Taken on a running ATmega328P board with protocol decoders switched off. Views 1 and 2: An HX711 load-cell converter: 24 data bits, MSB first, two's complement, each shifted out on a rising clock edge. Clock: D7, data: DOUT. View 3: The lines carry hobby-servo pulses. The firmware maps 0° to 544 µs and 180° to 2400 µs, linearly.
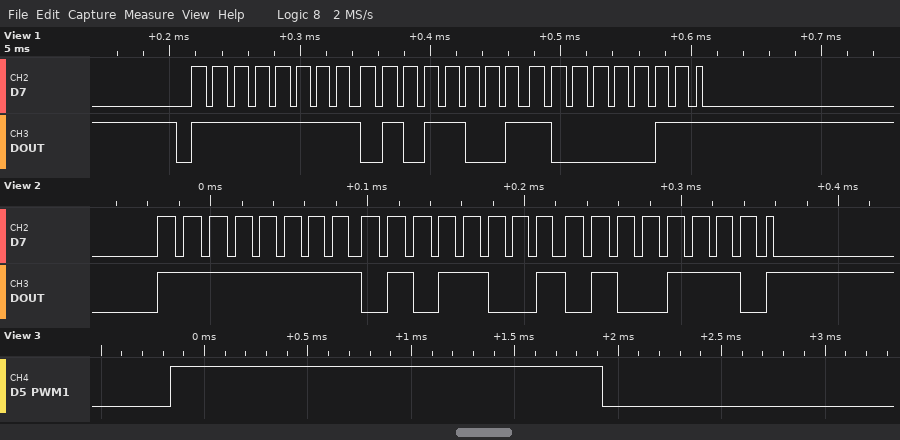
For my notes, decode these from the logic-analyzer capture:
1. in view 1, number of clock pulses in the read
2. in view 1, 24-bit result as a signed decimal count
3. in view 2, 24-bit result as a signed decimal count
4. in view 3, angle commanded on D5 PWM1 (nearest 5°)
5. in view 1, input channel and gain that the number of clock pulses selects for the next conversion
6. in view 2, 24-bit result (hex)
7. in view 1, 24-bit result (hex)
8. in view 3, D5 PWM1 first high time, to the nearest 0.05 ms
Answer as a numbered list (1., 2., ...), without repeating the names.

1. 25
2. -42621
3. -42674
4. 150°
5. channel A, gain 128
6. 0xFF594E
7. 0xFF5983
8. 2.10 ms
